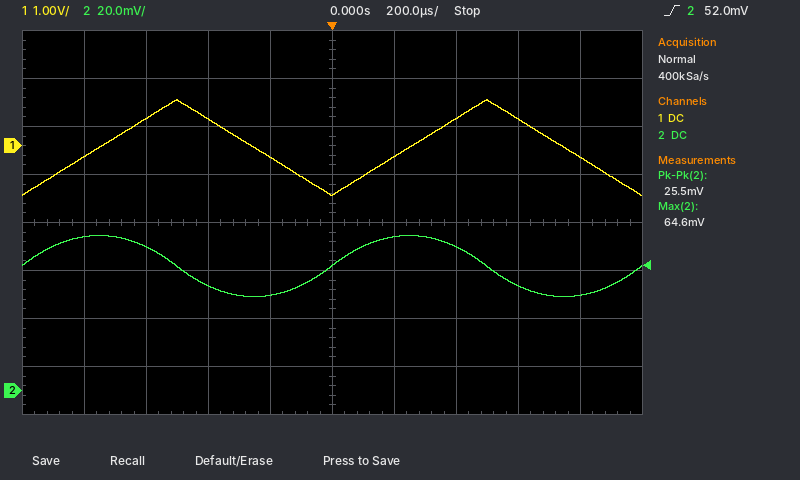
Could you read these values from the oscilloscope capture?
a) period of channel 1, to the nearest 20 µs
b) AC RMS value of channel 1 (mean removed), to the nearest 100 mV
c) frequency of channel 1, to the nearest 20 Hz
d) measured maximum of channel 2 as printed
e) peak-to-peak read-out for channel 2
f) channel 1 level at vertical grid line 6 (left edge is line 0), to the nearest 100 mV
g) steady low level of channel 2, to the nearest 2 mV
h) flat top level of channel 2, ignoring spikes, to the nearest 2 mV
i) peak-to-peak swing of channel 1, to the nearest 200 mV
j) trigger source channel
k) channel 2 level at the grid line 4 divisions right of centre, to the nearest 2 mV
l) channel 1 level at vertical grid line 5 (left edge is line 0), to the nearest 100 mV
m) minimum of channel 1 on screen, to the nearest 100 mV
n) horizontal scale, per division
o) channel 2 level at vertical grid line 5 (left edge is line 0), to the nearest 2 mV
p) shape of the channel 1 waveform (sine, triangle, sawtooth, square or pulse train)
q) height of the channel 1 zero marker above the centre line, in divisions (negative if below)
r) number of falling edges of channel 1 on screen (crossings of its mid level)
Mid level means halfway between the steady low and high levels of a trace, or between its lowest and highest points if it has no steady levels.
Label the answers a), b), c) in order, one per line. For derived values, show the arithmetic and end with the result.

a) 1.00 ms
b) 2.0 V / (2√3) ≈ 577 mV, so 600 mV to the nearest 100 mV
c) 1 / 1.00 ms ≈ 1.00 kHz
d) 64.6 mV
e) 25.5 mV
f) -200 mV
g) 40 mV
h) 64 mV
i) 2.0 V
j) channel 2
k) 40 mV
l) -1.0 V
m) -1.0 V
n) 200 µs
o) 52 mV
p) triangle
q) +1.6 div
r) 2
